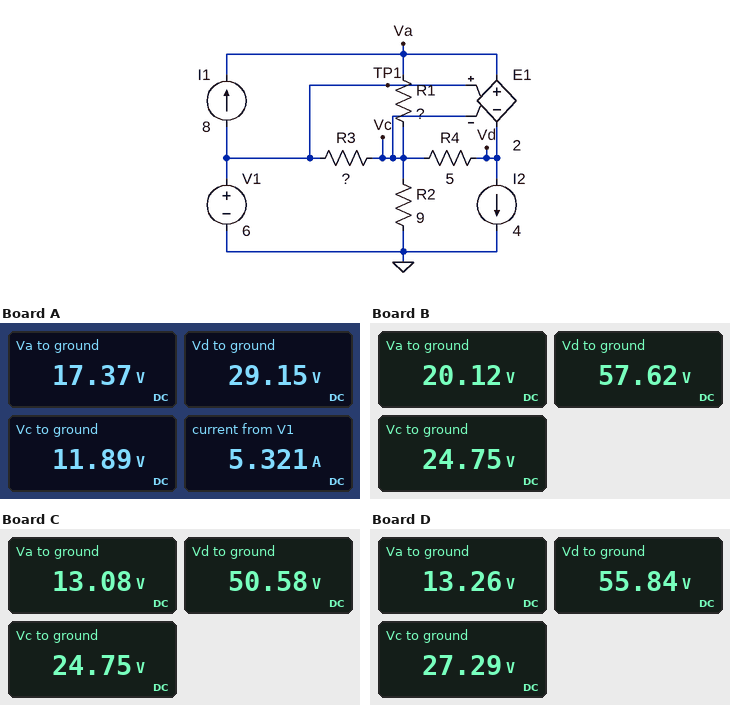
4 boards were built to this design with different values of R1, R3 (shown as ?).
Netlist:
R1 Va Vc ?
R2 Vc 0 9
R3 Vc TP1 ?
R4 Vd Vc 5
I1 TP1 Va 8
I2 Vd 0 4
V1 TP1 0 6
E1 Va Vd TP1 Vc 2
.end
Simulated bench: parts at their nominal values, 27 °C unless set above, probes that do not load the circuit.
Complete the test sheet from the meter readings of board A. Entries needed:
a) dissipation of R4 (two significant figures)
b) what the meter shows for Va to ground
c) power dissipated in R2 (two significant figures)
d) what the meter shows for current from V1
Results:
60 W
17.37 V
16 W
5.321 A
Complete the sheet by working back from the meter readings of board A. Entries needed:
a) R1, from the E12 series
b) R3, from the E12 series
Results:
10 Ω
2.2 Ω
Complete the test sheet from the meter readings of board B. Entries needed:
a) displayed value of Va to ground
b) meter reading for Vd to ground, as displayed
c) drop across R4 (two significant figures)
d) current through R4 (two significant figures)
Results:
20.12 V
57.62 V
33 V
6.6 A
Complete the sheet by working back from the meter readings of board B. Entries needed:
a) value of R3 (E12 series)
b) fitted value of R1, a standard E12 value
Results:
15 Ω
1.8 Ω
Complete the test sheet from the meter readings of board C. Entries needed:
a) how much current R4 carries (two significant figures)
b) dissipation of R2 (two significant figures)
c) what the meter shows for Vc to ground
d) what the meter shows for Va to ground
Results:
5.2 A
68 W
24.75 V
13.08 V
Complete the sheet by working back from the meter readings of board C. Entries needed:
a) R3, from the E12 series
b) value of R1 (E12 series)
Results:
15 Ω
10 Ω
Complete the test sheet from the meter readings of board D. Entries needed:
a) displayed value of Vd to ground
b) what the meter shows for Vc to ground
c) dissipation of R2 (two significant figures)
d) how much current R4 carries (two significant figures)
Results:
55.84 V
27.29 V
83 W
5.7 A
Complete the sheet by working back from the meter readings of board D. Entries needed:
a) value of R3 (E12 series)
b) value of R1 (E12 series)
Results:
22 Ω
8.2 Ω
